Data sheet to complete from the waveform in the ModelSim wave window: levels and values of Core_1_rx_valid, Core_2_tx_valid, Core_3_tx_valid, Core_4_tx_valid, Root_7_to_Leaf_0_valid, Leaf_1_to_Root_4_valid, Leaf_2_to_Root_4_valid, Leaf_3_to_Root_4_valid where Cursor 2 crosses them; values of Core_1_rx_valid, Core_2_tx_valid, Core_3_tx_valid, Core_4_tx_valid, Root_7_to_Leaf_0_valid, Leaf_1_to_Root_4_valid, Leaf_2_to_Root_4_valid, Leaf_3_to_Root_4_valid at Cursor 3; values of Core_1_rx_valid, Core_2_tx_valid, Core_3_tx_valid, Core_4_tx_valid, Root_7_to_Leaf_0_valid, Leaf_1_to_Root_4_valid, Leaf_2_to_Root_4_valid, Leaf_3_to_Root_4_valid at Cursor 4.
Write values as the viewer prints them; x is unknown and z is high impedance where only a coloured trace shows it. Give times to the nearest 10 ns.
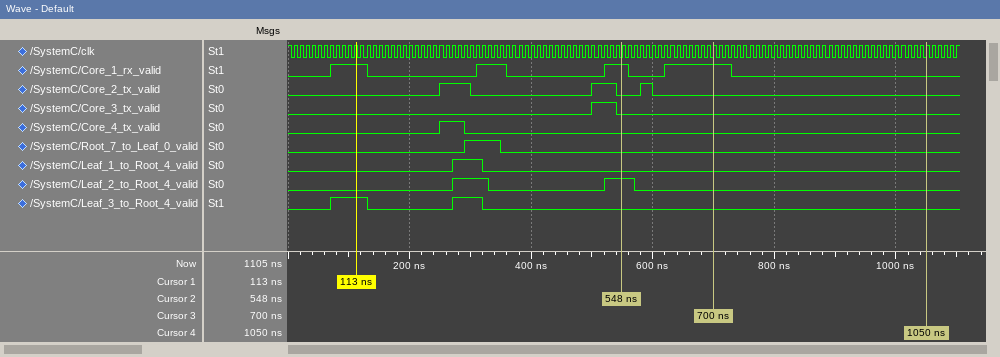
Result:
Core_1_rx_valid=1, Core_2_tx_valid=0, Core_3_tx_valid=0, Core_4_tx_valid=0, Root_7_to_Leaf_0_valid=0, Leaf_1_to_Root_4_valid=0, Leaf_2_to_Root_4_valid=1, Leaf_3_to_Root_4_valid=0
Core_1_rx_valid=1, Core_2_tx_valid=0, Core_3_tx_valid=0, Core_4_tx_valid=0, Root_7_to_Leaf_0_valid=0, Leaf_1_to_Root_4_valid=0, Leaf_2_to_Root_4_valid=0, Leaf_3_to_Root_4_valid=0
Core_1_rx_valid=0, Core_2_tx_valid=0, Core_3_tx_valid=0, Core_4_tx_valid=0, Root_7_to_Leaf_0_valid=0, Leaf_1_to_Root_4_valid=0, Leaf_2_to_Root_4_valid=0, Leaf_3_to_Root_4_valid=0
